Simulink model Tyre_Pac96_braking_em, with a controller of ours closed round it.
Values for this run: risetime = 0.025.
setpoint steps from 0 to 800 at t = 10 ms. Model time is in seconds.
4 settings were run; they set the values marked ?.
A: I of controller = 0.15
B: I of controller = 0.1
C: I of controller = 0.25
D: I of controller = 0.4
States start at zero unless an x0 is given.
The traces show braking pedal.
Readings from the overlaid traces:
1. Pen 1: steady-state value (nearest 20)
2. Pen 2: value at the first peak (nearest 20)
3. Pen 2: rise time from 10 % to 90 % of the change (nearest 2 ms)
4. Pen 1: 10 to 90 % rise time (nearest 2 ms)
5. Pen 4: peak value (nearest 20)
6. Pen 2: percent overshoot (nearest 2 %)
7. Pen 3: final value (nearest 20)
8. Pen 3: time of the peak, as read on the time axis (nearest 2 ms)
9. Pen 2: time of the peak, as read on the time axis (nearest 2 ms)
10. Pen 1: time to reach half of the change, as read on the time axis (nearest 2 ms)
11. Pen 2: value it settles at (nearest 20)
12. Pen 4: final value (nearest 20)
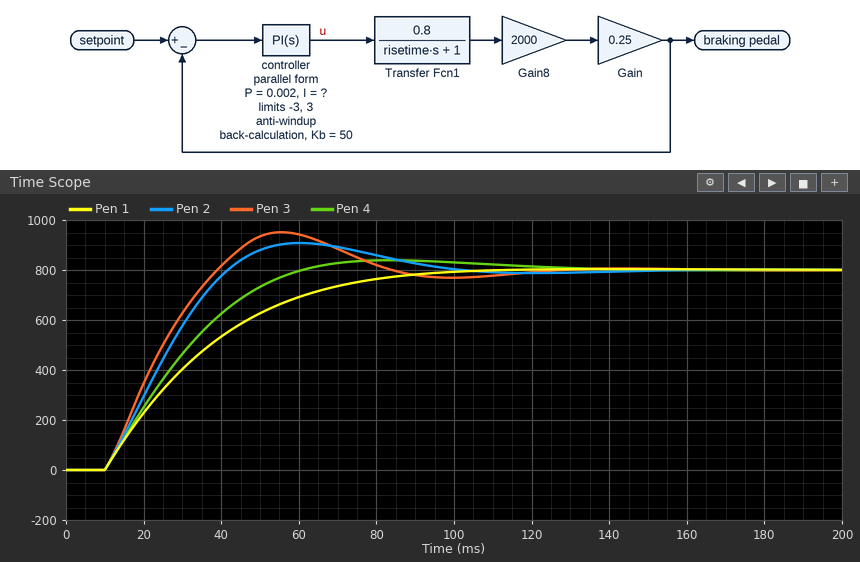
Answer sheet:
800
900
24 ms
52 ms
840
14 %
800
56 ms
60 ms
30 ms
800
800
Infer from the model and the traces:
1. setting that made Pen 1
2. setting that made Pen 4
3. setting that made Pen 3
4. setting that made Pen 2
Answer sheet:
B
A
D
C
